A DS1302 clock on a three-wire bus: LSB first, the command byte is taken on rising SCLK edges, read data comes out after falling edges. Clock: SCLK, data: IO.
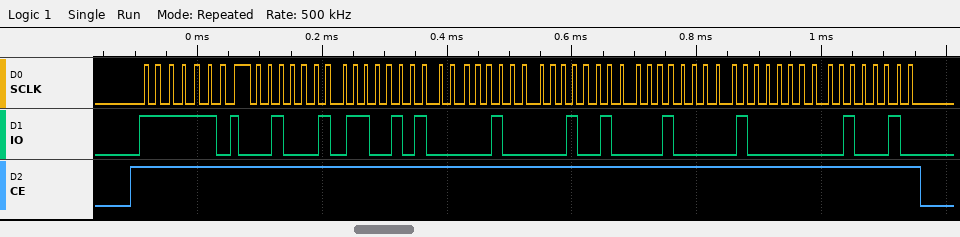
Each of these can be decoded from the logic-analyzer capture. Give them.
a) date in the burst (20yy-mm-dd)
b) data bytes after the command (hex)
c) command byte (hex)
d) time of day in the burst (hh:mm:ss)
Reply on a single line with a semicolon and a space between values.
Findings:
2022-04-24; 44 53 10 24 04 01 22; 0xBF; 10:53:44
